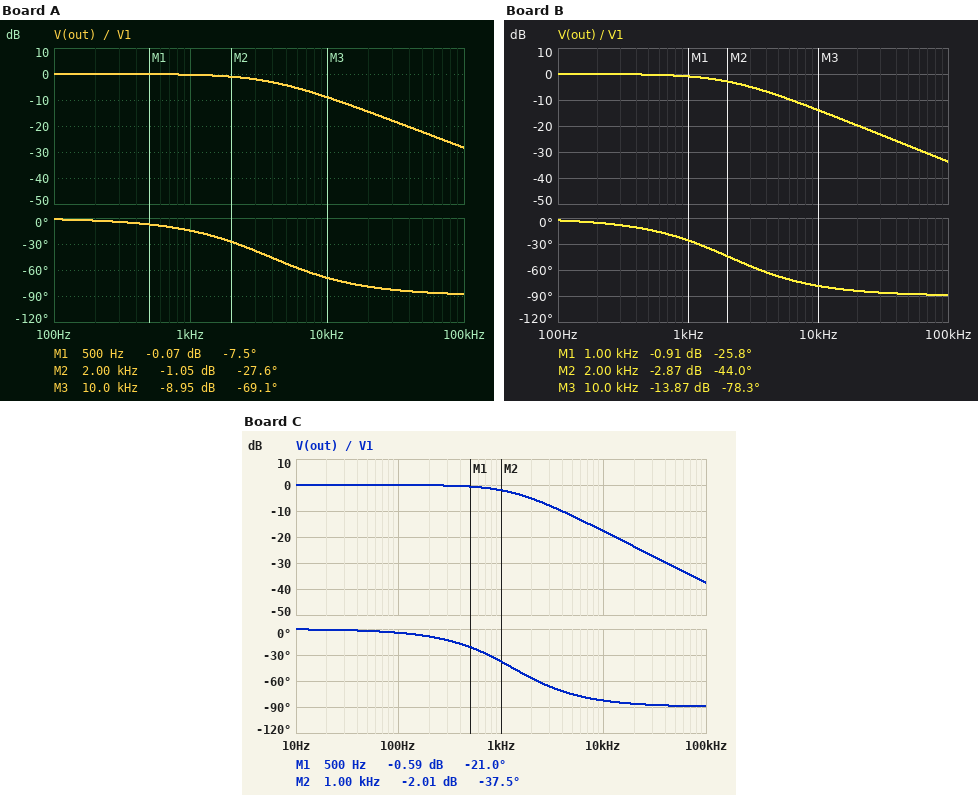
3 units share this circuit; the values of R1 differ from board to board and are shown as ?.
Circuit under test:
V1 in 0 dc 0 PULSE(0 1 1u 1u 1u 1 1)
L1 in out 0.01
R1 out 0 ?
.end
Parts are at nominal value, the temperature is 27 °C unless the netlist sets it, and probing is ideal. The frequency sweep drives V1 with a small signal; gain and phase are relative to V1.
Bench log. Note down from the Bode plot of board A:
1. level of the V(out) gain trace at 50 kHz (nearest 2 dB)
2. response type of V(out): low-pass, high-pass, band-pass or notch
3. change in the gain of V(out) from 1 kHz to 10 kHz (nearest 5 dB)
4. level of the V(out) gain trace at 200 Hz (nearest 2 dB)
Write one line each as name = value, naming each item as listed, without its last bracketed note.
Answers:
level of the V(out) gain trace at 50 kHz = -22 dB
response type of V(out): low-pass, high-pass, band-pass or notch = low-pass
change in the gain of V(out) from 1 kHz to 10 kHz = -10 dB
level of the V(out) gain trace at 200 Hz = 0 dB
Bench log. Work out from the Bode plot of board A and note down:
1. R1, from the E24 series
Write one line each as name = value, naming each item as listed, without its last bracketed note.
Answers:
R1, from the E24 series = 240 Ω
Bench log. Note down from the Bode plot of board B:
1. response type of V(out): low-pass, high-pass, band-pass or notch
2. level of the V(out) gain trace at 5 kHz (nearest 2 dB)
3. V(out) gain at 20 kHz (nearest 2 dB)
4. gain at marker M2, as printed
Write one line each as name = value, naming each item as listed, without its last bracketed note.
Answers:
response type of V(out): low-pass, high-pass, band-pass or notch = low-pass
level of the V(out) gain trace at 5 kHz = -8 dB
V(out) gain at 20 kHz = -20 dB
gain at marker M2, as printed = -2.87 dB
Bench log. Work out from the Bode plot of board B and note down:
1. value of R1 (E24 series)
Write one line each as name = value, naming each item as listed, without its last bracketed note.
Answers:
value of R1 = 130 Ω
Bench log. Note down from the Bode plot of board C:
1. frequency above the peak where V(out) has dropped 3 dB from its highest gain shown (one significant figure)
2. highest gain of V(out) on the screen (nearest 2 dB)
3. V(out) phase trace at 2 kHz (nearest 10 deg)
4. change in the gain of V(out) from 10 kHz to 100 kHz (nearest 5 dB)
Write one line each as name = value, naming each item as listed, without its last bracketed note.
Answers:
frequency above the peak where V(out) has dropped 3 dB from its highest gain shown = 1 kHz
highest gain of V(out) on the screen = 0 dB
V(out) phase trace at 2 kHz = -60 deg
change in the gain of V(out) from 10 kHz to 100 kHz = -20 dB
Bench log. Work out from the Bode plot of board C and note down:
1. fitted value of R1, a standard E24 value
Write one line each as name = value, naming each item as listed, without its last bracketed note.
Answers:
fitted value of R1, a standard E24 value = 82 Ω
